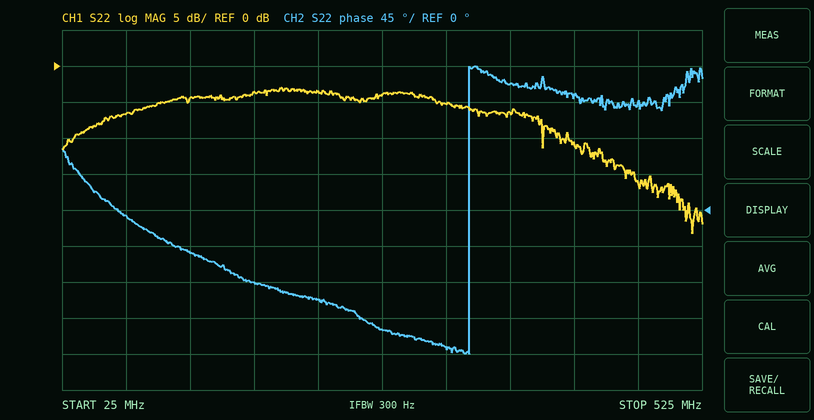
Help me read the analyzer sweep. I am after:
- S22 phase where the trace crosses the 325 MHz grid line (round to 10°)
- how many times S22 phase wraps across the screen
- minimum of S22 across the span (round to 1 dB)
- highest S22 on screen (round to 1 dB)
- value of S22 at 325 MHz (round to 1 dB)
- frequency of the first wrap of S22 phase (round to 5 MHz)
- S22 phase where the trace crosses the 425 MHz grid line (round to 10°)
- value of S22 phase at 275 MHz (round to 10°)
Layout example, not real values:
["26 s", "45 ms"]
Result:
["-170°", "1", "-23 dB", "-3 dB", "-5 dB", "345 MHz", "140°", "-150°"]
